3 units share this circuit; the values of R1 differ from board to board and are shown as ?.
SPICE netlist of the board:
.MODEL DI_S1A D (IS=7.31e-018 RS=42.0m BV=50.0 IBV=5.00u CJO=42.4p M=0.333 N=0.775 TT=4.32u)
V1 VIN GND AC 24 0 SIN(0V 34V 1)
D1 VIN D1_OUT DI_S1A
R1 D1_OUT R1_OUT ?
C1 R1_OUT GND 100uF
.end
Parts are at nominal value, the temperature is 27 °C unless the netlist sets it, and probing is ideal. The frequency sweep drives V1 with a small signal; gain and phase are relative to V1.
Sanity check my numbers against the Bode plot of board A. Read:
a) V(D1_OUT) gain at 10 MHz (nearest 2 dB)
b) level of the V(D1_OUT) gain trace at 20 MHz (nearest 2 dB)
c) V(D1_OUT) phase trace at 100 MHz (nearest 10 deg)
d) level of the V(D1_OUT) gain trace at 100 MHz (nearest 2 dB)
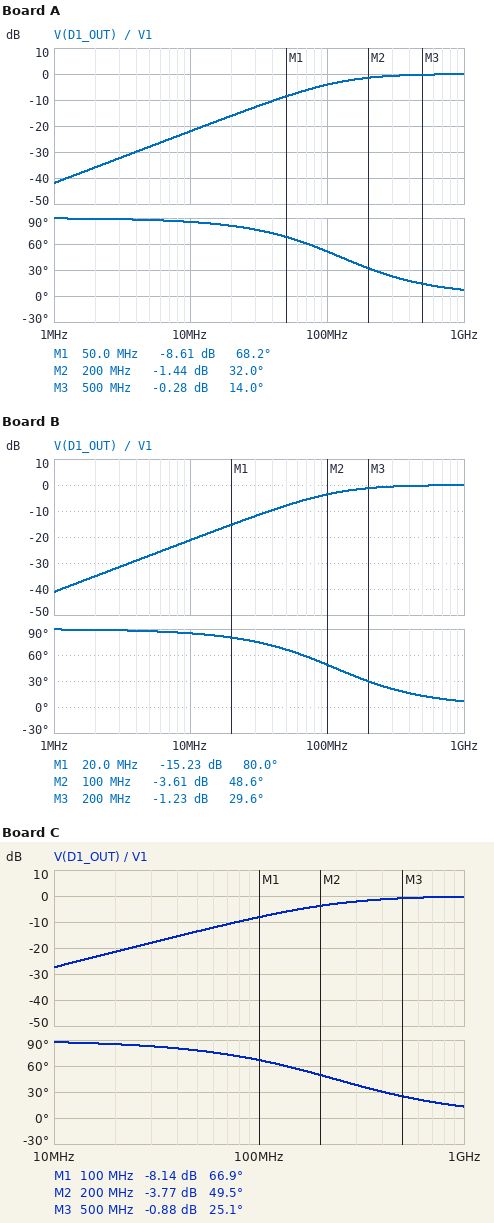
-22 dB
-16 dB
50 deg
-4 dB
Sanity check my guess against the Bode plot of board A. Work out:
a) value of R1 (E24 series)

30 Ω
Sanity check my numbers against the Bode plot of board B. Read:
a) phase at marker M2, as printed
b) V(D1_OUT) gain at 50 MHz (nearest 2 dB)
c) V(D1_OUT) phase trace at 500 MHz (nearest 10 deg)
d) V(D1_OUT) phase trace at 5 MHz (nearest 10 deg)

48.6 deg
-8 dB
10 deg
90 deg
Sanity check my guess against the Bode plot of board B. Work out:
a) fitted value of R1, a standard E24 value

33 Ω
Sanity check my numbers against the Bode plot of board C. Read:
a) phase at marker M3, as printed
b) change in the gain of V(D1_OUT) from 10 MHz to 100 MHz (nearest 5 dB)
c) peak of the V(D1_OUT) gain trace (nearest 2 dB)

25.1 deg
20 dB
0 dB
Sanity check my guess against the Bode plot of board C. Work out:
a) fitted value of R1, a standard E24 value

16 Ω
